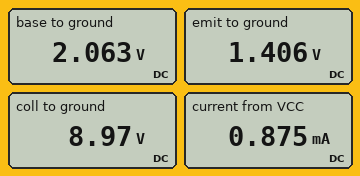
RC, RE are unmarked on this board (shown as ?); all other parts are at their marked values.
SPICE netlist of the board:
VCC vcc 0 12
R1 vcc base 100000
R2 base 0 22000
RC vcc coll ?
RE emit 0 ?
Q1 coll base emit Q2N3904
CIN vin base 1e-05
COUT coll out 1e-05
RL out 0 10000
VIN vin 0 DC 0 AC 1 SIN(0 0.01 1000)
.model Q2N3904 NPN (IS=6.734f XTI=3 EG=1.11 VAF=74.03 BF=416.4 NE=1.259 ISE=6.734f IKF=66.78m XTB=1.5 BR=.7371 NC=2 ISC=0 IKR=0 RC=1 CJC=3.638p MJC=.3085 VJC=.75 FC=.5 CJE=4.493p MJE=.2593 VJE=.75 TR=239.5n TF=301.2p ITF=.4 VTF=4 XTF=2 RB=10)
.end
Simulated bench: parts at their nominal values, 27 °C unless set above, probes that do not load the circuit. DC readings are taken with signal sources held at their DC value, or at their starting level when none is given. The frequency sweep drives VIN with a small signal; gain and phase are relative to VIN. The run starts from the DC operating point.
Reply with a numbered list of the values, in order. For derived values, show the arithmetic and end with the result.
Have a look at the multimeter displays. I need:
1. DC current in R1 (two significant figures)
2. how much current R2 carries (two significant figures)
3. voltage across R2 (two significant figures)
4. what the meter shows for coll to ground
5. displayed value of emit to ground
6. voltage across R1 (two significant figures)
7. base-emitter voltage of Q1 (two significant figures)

1. (12 V - 2.063 V) / 100 kΩ = 99 µA
2. (2.063 V) / 22 kΩ = 94 µA
3. 2.063 V = 2.1 V
4. 8.97 V
5. 1.406 V
6. 12 V - 2.063 V = 9.9 V
7. 2.063 V - 1.406 V = 660 mV
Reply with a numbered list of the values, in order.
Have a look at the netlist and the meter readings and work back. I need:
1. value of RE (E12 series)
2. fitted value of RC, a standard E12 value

1. 1.8 kΩ
2. 3.9 kΩ
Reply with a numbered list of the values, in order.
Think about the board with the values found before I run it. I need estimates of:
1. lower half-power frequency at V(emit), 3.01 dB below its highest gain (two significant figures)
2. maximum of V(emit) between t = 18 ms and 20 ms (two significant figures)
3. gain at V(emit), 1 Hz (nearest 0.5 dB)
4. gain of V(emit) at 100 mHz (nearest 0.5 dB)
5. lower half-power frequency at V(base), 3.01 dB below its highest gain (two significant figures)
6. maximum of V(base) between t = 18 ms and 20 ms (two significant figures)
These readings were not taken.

1. 940 mHz
2. 1.4 V
3. -3.0 dB
4. -19.5 dB
5. 940 mHz
6. 2.1 V
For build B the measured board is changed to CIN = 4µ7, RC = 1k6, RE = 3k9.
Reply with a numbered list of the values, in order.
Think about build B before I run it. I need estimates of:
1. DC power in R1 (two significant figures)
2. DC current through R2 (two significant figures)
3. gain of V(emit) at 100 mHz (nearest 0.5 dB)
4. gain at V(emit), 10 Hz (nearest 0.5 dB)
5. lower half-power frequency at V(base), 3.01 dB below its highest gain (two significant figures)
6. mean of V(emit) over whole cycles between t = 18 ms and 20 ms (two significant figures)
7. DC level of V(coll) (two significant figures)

1. 980 µW
2. 96 µA
3. -26.0 dB
4. -0.5 dB
5. 1.9 Hz
6. 1.5 V
7. 11 V
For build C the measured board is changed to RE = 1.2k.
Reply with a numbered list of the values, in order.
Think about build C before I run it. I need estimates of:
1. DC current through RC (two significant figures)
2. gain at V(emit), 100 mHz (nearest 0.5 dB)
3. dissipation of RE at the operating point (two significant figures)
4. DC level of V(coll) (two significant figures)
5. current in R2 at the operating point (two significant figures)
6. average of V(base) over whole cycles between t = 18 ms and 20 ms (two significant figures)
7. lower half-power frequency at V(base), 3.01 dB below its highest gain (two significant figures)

1. 1.1 mA
2. -20.0 dB
3. 1.5 mW
4. 7.6 V
5. 92 µA
6. 2.0 V
7. 970 mHz
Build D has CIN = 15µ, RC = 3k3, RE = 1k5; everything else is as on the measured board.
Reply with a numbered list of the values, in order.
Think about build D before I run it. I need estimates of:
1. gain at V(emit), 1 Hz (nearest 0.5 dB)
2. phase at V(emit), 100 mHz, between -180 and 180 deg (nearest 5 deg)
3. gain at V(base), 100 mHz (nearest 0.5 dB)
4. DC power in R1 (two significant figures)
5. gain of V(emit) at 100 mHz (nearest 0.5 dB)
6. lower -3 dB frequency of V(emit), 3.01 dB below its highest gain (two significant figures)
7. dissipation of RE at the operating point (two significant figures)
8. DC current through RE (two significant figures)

1. -1.5 dB
2. 80 deg
3. -16.0 dB
4. 990 µW
5. -16.5 dB
6. 630 mHz
7. 1.3 mW
8. 920 µA
